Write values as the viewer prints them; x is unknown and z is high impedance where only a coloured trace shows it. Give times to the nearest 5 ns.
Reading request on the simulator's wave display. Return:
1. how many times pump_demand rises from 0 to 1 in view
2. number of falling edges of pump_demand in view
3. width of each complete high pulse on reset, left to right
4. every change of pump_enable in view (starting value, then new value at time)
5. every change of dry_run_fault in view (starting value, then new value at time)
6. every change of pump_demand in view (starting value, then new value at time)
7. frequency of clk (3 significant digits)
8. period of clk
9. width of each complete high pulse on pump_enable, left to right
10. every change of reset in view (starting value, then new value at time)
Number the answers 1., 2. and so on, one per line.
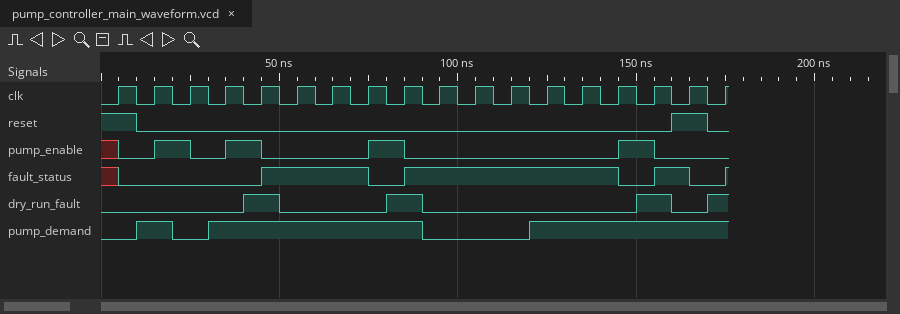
1. 3
2. 2
3. 10 ns
4. x, 0 at 5 ns, 1 at 15 ns, 0 at 25 ns, 1 at 35 ns, 0 at 45 ns, 1 at 75 ns, 0 at 85 ns, 1 at 145 ns, 0 at 155 ns
5. 0, 1 at 40 ns, 0 at 50 ns, 1 at 80 ns, 0 at 90 ns, 1 at 150 ns, 0 at 160 ns, 1 at 170 ns
6. 0, 1 at 10 ns, 0 at 20 ns, 1 at 30 ns, 0 at 90 ns, 1 at 120 ns
7. 100 MHz
8. 10 ns
9. 10 ns, 10 ns, 10 ns, 10 ns
10. 1, 0 at 10 ns, 1 at 160 ns, 0 at 170 ns
